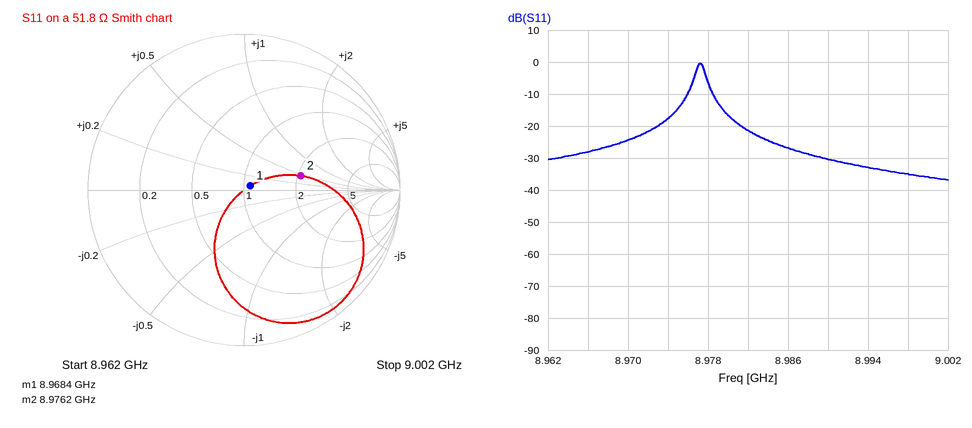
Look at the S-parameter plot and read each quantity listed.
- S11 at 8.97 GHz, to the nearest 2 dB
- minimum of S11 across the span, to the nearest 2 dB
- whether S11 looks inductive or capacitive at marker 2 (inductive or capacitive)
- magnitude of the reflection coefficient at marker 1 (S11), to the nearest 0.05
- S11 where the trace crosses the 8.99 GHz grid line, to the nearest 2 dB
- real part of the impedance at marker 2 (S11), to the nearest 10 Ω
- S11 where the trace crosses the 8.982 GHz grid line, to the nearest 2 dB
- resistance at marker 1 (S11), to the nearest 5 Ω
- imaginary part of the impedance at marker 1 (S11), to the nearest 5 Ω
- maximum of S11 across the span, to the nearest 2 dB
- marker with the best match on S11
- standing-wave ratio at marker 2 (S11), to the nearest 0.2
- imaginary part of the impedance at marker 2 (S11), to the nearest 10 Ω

-24 dB
-36 dB
inductive
0.05
-30 dB
110 Ω
-22 dB
55 Ω
+5 Ω
0 dB
marker 1
2.2
+20 Ω
